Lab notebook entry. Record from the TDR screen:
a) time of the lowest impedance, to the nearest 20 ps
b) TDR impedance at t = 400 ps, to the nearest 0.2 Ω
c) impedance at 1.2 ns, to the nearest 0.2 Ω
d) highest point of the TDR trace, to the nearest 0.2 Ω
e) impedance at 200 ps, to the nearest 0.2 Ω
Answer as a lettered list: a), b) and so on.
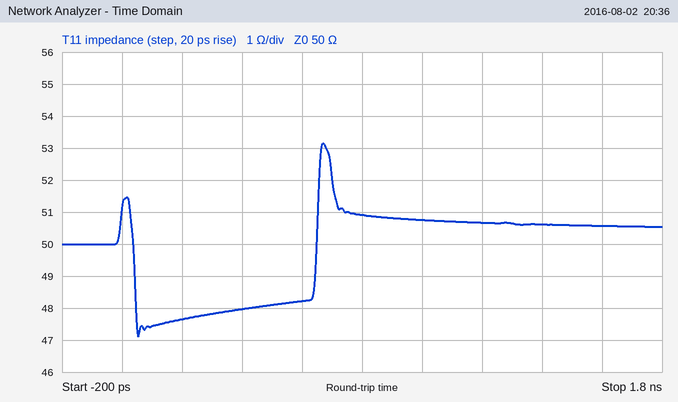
a) 60 ps
b) 48.0 Ω
c) 50.6 Ω
d) 53.2 Ω
e) 47.6 Ω
